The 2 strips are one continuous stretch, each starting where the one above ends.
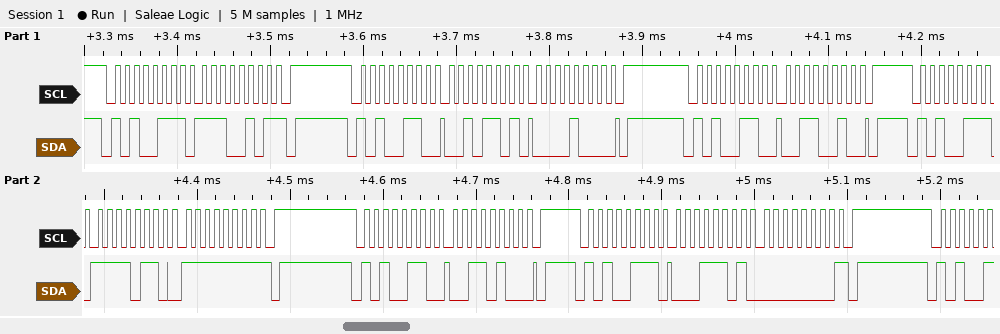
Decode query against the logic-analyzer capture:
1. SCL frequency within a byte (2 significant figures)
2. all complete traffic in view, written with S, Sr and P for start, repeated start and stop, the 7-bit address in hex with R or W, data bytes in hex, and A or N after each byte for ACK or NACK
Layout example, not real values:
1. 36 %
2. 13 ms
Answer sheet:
1. 100 kHz
2. S 53R A E5 N P S 53W A 2D A 08 A P S 53W A 32 A P S 53R A F6 A FF N P S 53W A 34 A P S 53R A 1D A 00 N P
